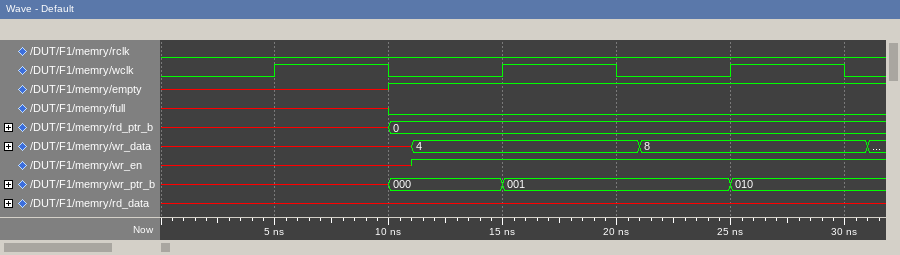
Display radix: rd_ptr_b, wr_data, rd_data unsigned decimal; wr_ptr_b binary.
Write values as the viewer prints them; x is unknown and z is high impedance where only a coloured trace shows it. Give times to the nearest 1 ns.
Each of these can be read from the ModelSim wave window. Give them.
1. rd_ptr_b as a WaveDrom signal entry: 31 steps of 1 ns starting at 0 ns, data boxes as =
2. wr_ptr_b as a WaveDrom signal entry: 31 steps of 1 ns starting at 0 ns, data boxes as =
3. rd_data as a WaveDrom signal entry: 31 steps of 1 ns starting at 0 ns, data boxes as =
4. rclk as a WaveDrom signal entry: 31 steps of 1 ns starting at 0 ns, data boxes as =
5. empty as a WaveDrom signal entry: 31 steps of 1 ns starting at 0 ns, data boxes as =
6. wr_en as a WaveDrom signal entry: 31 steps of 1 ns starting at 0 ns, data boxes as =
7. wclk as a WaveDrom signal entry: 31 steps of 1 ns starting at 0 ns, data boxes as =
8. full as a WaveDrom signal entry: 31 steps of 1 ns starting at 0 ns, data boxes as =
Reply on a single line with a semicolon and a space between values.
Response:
{name: 'rd_ptr_b', wave: 'x.........=....................', data: '0'}; {name: 'wr_ptr_b', wave: 'x.........=....=.........=.....', data: '000 001 010'}; {name: 'rd_data', wave: 'x..............................'}; {name: 'rclk', wave: '0..............................'}; {name: 'empty', wave: 'x.........1....................'}; {name: 'wr_en', wave: 'x..........1...................'}; {name: 'wclk', wave: '0....1....0....1....0....1....0'}; {name: 'full', wave: 'x.........0....................'}
